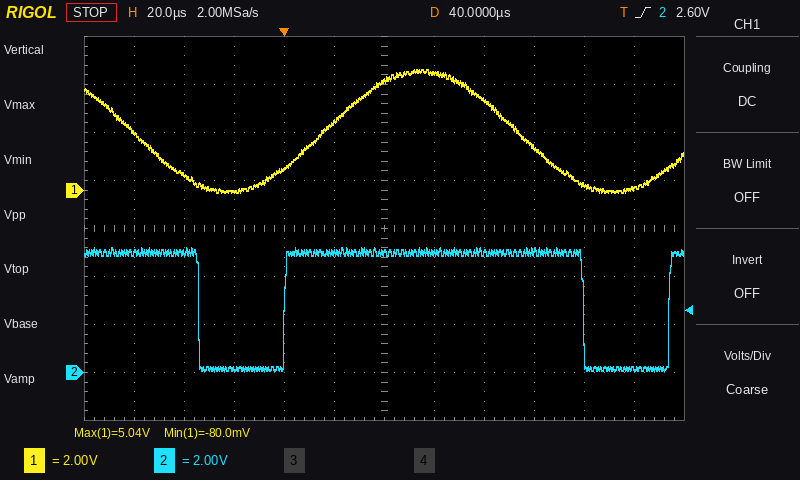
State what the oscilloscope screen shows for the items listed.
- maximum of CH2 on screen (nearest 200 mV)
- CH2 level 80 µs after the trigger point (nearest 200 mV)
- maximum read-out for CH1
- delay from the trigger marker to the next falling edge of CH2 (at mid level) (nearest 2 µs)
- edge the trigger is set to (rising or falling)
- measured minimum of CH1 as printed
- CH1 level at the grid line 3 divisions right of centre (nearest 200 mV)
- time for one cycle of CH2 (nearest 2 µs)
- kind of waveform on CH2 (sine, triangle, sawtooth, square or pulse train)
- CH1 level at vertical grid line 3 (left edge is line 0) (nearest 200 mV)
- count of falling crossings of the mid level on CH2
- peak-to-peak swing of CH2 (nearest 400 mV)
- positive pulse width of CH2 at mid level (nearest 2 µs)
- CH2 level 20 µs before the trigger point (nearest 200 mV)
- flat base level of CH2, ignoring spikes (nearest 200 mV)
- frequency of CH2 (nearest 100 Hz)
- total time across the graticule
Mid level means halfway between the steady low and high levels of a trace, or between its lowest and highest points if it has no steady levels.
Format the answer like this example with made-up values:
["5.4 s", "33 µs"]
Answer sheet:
["5.2 V", "5.0 V", "5.04 V", "120 µs", "rising", "-80.0 mV", "1.8 V", "154 µs", "pulse train", "0.0 V", "2", "5.2 V", "120 µs", "200 mV", "200 mV", "6.5 kHz", "240 µs"]
